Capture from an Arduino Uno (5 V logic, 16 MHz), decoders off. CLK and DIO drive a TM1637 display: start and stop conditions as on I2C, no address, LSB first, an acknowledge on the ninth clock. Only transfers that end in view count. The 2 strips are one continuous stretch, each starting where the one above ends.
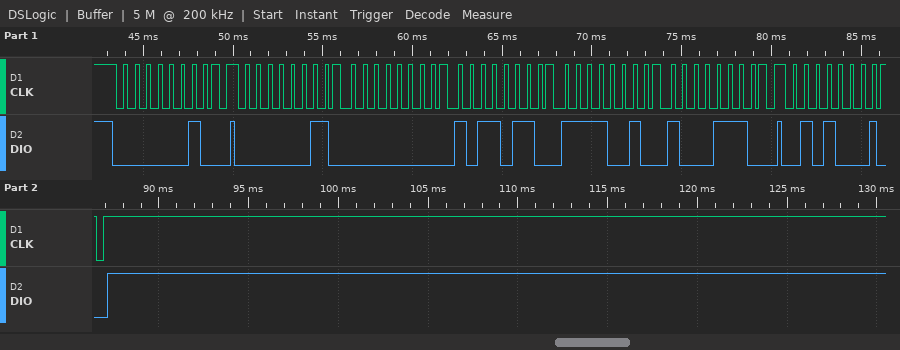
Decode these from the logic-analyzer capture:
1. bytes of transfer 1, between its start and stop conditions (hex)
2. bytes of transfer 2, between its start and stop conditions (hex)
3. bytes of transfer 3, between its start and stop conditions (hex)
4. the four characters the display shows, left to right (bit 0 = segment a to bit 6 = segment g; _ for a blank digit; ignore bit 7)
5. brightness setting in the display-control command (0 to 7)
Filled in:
40
C0 00 6D 4F 71
8A
_53F
2
